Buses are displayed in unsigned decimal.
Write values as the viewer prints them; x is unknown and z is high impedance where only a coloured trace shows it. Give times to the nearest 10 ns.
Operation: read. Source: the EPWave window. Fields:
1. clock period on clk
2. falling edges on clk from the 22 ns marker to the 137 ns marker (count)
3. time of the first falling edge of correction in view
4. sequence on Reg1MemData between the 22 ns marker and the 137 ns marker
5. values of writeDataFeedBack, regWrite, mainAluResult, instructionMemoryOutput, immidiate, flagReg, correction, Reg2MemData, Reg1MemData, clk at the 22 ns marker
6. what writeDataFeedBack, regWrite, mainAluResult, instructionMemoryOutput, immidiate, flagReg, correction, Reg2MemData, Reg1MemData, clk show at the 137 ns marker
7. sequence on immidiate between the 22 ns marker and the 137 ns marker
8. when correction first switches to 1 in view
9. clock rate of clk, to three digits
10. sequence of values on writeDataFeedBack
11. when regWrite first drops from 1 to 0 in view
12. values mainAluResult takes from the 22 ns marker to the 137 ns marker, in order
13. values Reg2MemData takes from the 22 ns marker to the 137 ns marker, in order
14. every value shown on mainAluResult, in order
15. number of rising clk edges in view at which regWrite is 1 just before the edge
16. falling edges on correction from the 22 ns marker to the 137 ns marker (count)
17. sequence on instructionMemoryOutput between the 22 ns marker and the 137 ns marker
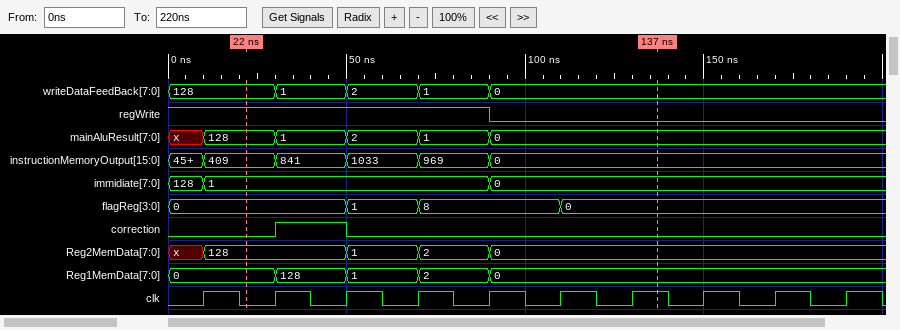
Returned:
20 ns
5
50 ns
0, 128, 1, 2, 0
writeDataFeedBack=128, regWrite=1, mainAluResult=128, instructionMemoryOutput=409, immidiate=1, flagReg=0, correction=0, Reg2MemData=128, Reg1MemData=0, clk=0
writeDataFeedBack=0, regWrite=0, mainAluResult=0, instructionMemoryOutput=0, immidiate=0, flagReg=0, correction=0, Reg2MemData=0, Reg1MemData=0, clk=1
1, 0
30 ns
50.0 MHz
128, 1, 2, 1, 0
90 ns
128, 1, 2, 1, 0
128, 1, 2, 0
x, 128, 1, 2, 1, 0
5
1
409, 841, 1033, 969, 0
